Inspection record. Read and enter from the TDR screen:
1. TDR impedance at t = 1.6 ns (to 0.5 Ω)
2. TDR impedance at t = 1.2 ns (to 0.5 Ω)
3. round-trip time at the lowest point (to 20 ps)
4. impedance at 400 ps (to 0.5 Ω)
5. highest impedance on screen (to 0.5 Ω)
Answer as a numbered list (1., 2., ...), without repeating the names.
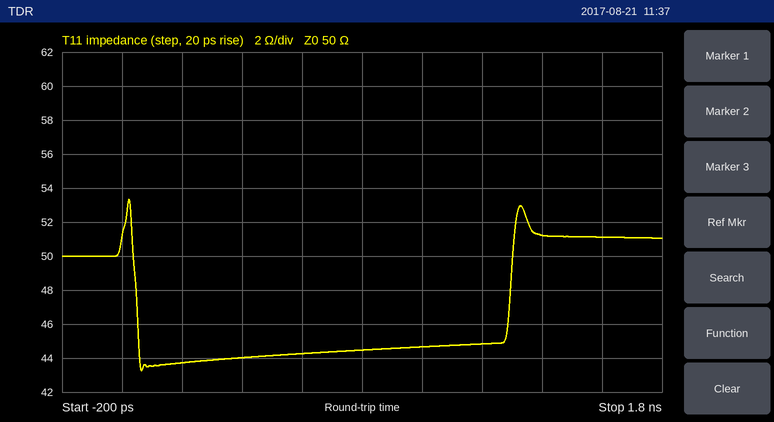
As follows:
1. 51.0 Ω
2. 45.0 Ω
3. 60 ps
4. 44.0 Ω
5. 53.5 Ω
